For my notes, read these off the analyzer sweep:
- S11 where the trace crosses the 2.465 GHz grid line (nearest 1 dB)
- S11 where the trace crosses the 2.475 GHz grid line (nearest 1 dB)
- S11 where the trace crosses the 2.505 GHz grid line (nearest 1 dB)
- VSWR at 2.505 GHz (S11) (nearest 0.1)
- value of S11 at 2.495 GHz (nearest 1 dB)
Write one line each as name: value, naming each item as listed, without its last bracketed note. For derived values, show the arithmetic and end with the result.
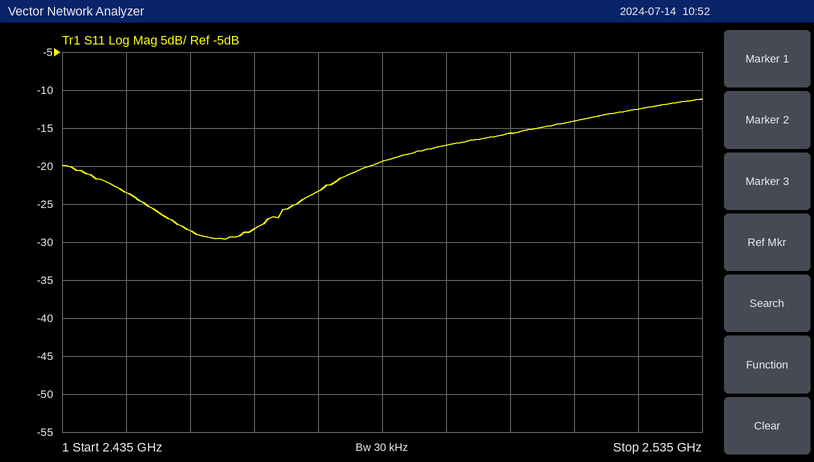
S11 where the trace crosses the 2.465 GHz grid line: -28 dB
S11 where the trace crosses the 2.475 GHz grid line: -23 dB
S11 where the trace crosses the 2.505 GHz grid line: -16 dB
VSWR at 2.505 GHz (S11): |Γ| = 10^(-16/20) = 0.1585; VSWR = (1 + 0.1585)/(1 − 0.1585) ≈ 1.4
value of S11 at 2.495 GHz: -17 dB
